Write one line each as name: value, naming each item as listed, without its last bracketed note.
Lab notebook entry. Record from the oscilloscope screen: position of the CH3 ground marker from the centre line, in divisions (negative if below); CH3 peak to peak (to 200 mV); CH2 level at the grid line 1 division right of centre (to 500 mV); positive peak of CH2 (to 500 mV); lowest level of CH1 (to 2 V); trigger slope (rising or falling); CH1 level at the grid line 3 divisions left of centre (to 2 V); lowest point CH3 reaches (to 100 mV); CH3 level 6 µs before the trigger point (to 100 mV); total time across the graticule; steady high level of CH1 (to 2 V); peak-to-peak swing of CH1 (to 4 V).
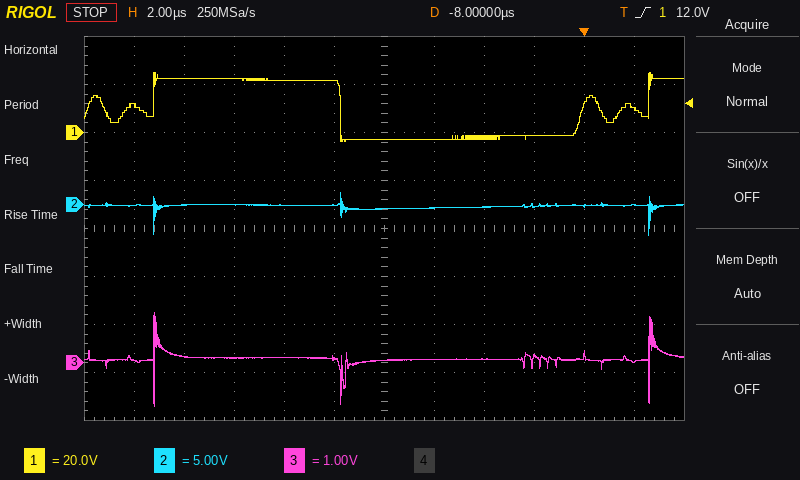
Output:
position of the CH3 ground marker from the centre line, in divisions: -2.8 div
CH3 peak to peak: 2.0 V
CH2 level at the grid line 1 division right of centre: -500 mV
positive peak of CH2: 1.0 V
lowest level of CH1: -4 V
trigger slope: rising
CH1 level at the grid line 3 divisions left of centre: 22 V
lowest point CH3 reaches: -900 mV
CH3 level 6 µs before the trigger point: 100 mV
total time across the graticule: 24 µs
steady high level of CH1: 22 V
peak-to-peak swing of CH1: 28 V
